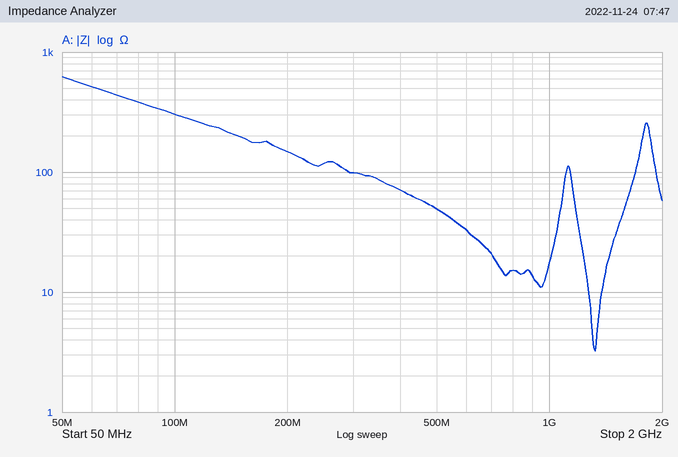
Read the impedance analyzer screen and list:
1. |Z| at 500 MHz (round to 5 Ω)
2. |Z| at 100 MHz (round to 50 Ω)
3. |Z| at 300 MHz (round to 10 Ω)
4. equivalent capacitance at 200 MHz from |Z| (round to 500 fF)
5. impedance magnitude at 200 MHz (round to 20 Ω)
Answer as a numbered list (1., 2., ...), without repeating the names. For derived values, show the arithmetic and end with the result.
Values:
1. 50 Ω
2. 300 Ω
3. 100 Ω
4. C = 1/(2π × 200 MHz × 140 Ω) ≈ 5.68 pF, so 5.5 pF to the nearest 500 fF
5. 140 Ω
